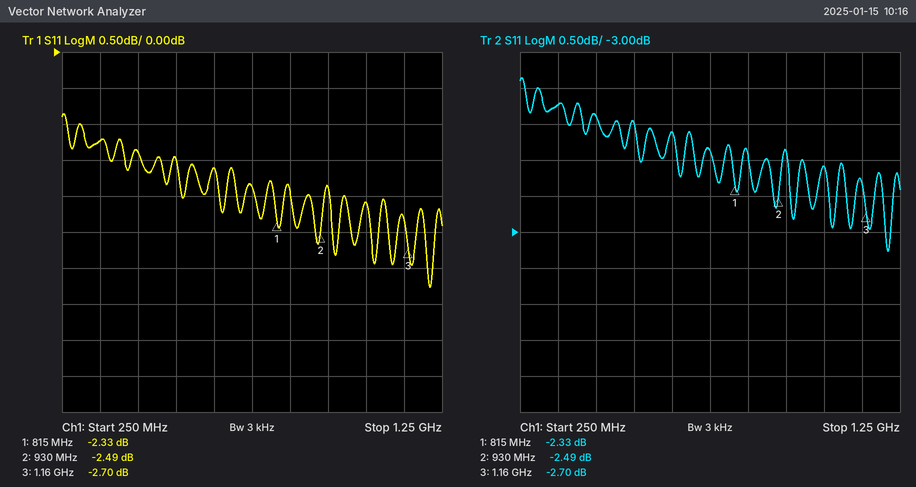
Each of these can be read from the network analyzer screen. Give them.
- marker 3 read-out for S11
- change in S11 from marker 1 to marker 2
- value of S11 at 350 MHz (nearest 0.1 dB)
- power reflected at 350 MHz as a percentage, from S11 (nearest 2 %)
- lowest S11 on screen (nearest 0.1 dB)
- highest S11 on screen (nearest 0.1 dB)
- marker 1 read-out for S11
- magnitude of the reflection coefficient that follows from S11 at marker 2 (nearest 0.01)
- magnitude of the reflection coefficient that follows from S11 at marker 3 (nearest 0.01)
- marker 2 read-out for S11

-2.70 dB
-0.16 dB
-1.2 dB
76 %
-3.3 dB
-0.9 dB
-2.33 dB
0.75
0.73
-2.49 dB
